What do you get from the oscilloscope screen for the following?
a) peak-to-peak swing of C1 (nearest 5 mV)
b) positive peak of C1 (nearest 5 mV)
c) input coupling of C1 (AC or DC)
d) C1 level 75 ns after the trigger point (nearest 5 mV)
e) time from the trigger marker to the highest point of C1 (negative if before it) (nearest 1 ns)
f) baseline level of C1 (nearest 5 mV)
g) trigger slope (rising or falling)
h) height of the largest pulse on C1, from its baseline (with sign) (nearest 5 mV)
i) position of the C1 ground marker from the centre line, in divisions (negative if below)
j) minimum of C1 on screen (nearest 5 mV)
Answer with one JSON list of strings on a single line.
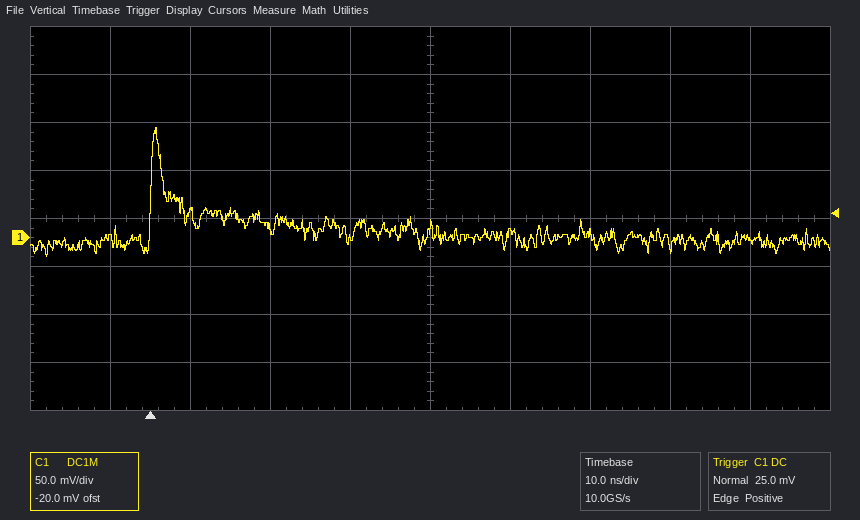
["135 mV", "115 mV", "DC", "0 mV", "+1 ns", "0 mV", "rising", "+115 mV", "-0.4 div", "-20 mV"]
